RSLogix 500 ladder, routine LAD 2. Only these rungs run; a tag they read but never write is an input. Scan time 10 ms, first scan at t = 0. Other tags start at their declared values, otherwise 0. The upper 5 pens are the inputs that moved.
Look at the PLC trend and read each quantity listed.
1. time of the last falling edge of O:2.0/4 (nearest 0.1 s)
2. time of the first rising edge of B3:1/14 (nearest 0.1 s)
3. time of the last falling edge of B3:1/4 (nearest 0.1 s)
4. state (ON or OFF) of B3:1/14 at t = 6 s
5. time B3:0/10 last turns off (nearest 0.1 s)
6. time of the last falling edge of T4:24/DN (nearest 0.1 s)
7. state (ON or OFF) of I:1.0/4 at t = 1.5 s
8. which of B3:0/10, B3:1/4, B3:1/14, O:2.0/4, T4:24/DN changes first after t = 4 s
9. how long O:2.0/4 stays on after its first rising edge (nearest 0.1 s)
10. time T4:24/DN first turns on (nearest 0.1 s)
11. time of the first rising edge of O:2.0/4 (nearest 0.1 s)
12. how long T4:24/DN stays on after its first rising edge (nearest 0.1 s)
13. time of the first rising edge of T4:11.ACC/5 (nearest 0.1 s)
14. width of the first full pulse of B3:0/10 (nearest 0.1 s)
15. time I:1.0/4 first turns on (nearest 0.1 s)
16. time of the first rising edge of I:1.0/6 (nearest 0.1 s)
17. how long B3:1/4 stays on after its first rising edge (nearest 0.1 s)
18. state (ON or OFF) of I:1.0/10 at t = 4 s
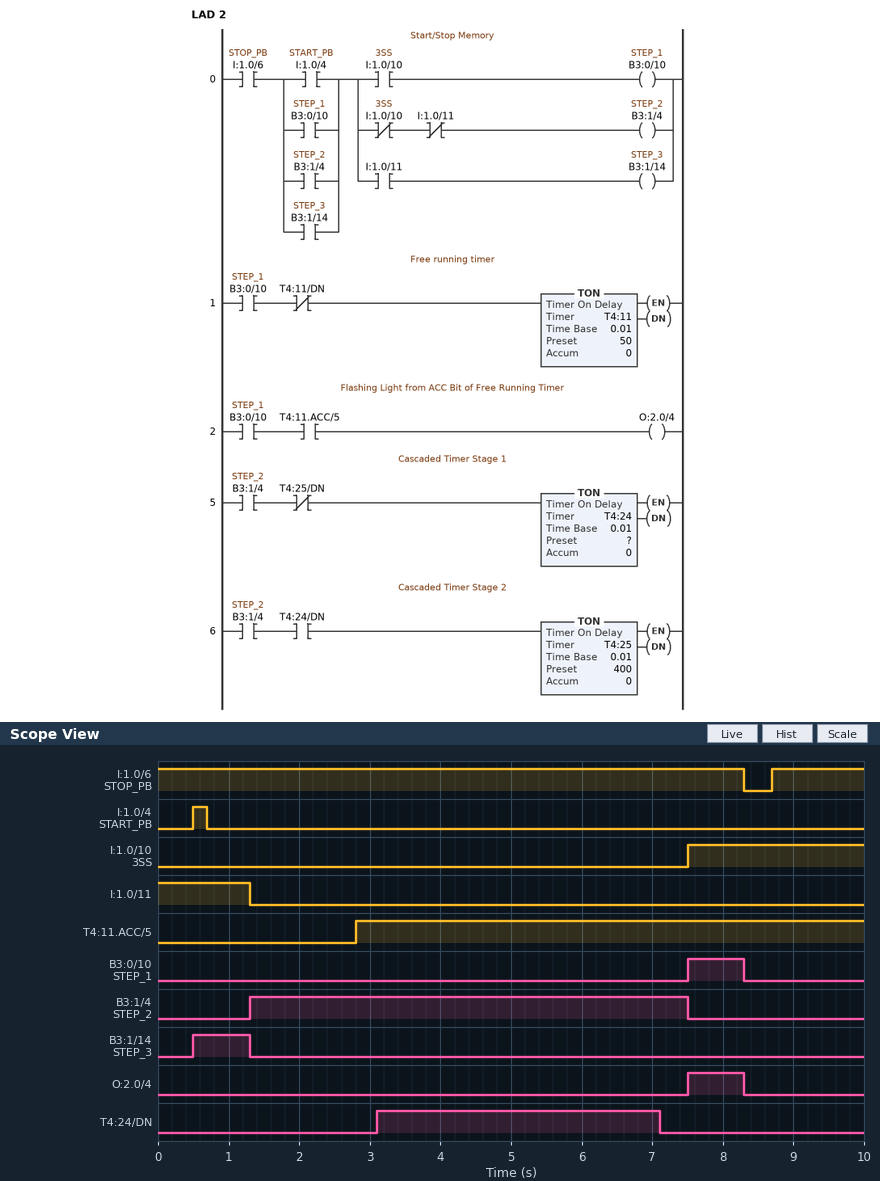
8.3 s
0.5 s
7.5 s
OFF
8.3 s
7.1 s
OFF
T4:24/DN
0.8 s
3.1 s
7.5 s
4.0 s
2.8 s
0.8 s
0.5 s
8.7 s
6.2 s
OFF
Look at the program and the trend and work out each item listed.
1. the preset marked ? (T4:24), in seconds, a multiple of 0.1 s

1.8 s
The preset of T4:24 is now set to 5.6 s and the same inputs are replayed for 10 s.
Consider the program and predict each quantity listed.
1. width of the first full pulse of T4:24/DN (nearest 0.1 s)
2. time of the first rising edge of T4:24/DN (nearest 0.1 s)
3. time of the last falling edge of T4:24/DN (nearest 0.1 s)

0.6 s
6.9 s
7.5 s
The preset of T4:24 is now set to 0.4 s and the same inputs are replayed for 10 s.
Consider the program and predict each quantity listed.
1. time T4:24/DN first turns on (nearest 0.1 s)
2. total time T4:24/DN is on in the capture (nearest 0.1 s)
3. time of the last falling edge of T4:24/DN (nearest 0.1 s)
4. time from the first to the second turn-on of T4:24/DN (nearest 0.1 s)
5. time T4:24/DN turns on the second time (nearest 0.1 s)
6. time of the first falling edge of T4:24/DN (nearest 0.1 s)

1.7 s
5.4 s
7.5 s
4.4 s
6.1 s
5.7 s
